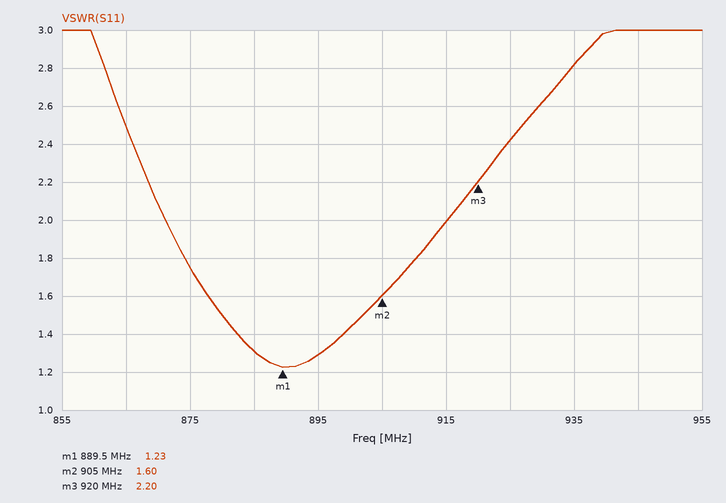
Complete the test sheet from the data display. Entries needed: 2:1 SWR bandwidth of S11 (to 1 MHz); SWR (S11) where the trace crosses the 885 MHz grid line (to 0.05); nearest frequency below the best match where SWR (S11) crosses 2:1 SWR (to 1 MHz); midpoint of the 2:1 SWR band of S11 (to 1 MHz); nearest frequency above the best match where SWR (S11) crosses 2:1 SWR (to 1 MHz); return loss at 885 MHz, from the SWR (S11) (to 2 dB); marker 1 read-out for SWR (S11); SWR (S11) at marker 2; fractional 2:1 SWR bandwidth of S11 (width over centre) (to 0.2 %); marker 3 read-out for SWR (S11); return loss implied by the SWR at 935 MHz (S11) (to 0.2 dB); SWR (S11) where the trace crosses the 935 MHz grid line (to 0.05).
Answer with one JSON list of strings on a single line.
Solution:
["44 MHz", "1.30", "871 MHz", "893 MHz", "915 MHz", "18 dB", "1.23", "1.60", "5.0 %", "2.20", "6.4 dB", "2.80"]
